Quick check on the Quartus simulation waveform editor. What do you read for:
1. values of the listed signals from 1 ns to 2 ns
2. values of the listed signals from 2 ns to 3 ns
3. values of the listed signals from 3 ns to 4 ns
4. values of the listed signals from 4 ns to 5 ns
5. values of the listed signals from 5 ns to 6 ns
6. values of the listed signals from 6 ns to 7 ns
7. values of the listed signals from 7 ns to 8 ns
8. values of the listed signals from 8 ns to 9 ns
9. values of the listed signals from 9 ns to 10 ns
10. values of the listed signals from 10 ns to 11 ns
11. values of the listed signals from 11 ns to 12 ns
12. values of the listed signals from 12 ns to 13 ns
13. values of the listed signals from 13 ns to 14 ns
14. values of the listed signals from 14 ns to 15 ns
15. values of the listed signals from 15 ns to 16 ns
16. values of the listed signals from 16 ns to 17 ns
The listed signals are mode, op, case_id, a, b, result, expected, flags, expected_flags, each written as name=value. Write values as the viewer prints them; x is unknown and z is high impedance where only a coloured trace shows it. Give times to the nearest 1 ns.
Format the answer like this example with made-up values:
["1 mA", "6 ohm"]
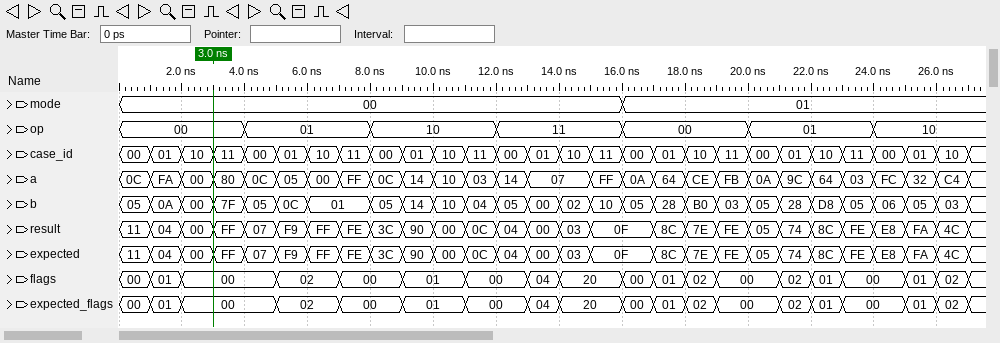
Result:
["mode=00, op=00, case_id=01, a=FA, b=0A, result=04, expected=04, flags=01, expected_flags=01", "mode=00, op=00, case_id=10, a=00, b=00, result=00, expected=00, flags=00, expected_flags=00", "mode=00, op=00, case_id=11, a=80, b=7F, result=FF, expected=FF, flags=00, expected_flags=00", "mode=00, op=01, case_id=00, a=0C, b=05, result=07, expected=07, flags=00, expected_flags=00", "mode=00, op=01, case_id=01, a=05, b=0C, result=F9, expected=F9, flags=02, expected_flags=02", "mode=00, op=01, case_id=10, a=00, b=01, result=FF, expected=FF, flags=02, expected_flags=02", "mode=00, op=01, case_id=11, a=FF, b=01, result=FE, expected=FE, flags=00, expected_flags=00", "mode=00, op=10, case_id=00, a=0C, b=05, result=3C, expected=3C, flags=00, expected_flags=00", "mode=00, op=10, case_id=01, a=14, b=14, result=90, expected=90, flags=01, expected_flags=01", "mode=00, op=10, case_id=10, a=10, b=10, result=00, expected=00, flags=01, expected_flags=01", "mode=00, op=10, case_id=11, a=03, b=04, result=0C, expected=0C, flags=00, expected_flags=00", "mode=00, op=11, case_id=00, a=14, b=05, result=04, expected=04, flags=00, expected_flags=00", "mode=00, op=11, case_id=01, a=07, b=00, result=00, expected=00, flags=04, expected_flags=04", "mode=00, op=11, case_id=10, a=07, b=02, result=03, expected=03, flags=20, expected_flags=20", "mode=00, op=11, case_id=11, a=FF, b=10, result=0F, expected=0F, flags=20, expected_flags=20", "mode=01, op=00, case_id=00, a=0A, b=05, result=0F, expected=0F, flags=00, expected_flags=00"]
